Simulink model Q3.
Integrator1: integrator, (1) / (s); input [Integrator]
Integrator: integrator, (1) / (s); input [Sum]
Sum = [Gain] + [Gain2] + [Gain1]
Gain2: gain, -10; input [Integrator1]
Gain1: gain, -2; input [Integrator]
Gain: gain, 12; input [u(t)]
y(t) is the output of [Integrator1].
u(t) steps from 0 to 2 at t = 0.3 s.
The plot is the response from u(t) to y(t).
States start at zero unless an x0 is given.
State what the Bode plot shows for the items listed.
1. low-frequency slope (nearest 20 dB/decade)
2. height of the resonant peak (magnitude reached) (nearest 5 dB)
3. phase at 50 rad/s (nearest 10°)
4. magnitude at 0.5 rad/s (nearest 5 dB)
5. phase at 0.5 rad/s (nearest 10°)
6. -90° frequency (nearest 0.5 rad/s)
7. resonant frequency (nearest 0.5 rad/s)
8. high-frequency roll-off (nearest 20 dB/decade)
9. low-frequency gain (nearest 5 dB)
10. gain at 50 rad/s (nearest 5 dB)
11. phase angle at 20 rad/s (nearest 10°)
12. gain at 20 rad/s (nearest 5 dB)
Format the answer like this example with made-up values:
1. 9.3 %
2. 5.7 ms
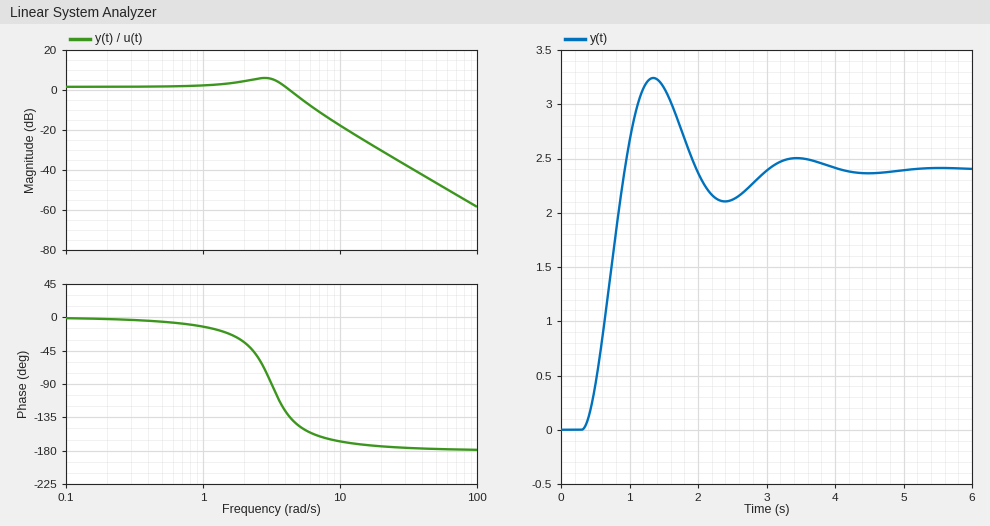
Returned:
1. 0 dB/decade
2. 5 dB
3. -180°
4. 0 dB
5. -10°
6. 3.0 rad/s
7. 3.0 rad/s
8. -40 dB/decade
9. 0 dB
10. -45 dB
11. -170°
12. -30 dB
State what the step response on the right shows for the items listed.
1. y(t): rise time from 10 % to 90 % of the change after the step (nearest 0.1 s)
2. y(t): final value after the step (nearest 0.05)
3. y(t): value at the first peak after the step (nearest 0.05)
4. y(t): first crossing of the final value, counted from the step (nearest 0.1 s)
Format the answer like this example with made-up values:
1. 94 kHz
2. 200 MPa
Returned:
1. 0.4 s
2. 2.40
3. 3.25
4. 0.6 s
